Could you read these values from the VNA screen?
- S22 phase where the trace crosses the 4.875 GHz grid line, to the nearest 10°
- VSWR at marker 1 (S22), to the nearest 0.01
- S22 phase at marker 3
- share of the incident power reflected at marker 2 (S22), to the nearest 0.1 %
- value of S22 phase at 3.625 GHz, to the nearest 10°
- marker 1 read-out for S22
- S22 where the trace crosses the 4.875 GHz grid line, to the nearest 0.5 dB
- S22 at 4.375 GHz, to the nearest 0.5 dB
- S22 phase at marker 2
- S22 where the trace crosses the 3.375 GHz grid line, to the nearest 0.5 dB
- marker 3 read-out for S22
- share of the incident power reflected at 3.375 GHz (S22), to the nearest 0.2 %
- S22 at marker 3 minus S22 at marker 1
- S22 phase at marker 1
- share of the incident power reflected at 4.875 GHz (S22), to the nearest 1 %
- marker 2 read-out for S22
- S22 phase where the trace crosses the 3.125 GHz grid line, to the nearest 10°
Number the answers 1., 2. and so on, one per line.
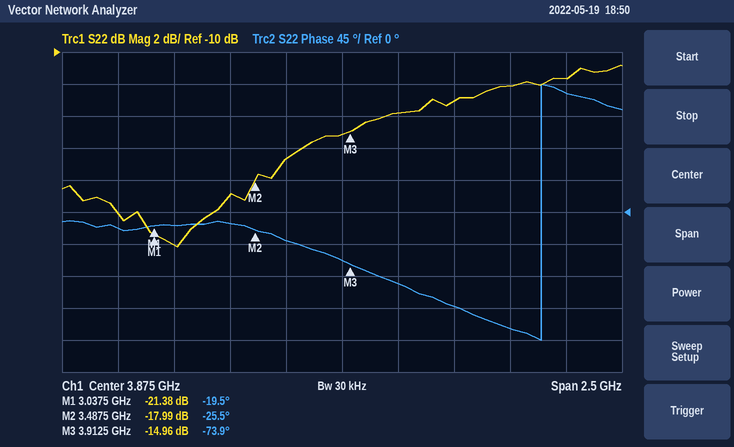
1. 170°
2. 1.19
3. -73.9°
4. 1.6 %
5. -40°
6. -21.38 dB
7. -11.5 dB
8. -13.0 dB
9. -25.5°
10. -19.0 dB
11. -14.96 dB
12. 1.2 %
13. 6.42 dB
14. -19.5°
15. 7 %
16. -17.99 dB
17. -20°
